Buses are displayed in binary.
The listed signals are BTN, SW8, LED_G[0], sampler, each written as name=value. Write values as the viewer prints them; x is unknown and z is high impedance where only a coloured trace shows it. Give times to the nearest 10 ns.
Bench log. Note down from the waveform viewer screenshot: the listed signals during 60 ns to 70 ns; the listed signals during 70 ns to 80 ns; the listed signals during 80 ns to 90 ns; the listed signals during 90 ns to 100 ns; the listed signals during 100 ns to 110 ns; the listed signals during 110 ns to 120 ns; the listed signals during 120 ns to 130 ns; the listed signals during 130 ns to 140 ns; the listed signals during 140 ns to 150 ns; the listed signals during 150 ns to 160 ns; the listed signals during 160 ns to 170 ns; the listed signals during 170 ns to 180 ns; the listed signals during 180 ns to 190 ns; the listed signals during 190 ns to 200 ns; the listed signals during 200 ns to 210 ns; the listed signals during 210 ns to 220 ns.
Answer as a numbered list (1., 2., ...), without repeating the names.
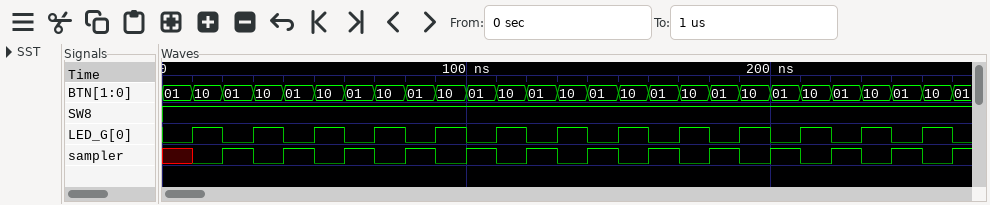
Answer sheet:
1. BTN=01, SW8=1, LED_G[0]=0, sampler=1
2. BTN=10, SW8=1, LED_G[0]=1, sampler=0
3. BTN=01, SW8=1, LED_G[0]=0, sampler=1
4. BTN=10, SW8=1, LED_G[0]=1, sampler=0
5. BTN=01, SW8=1, LED_G[0]=0, sampler=1
6. BTN=10, SW8=1, LED_G[0]=1, sampler=0
7. BTN=01, SW8=1, LED_G[0]=0, sampler=1
8. BTN=10, SW8=1, LED_G[0]=1, sampler=0
9. BTN=01, SW8=1, LED_G[0]=0, sampler=1
10. BTN=10, SW8=1, LED_G[0]=1, sampler=0
11. BTN=01, SW8=1, LED_G[0]=0, sampler=1
12. BTN=10, SW8=1, LED_G[0]=1, sampler=0
13. BTN=01, SW8=1, LED_G[0]=0, sampler=1
14. BTN=10, SW8=1, LED_G[0]=1, sampler=0
15. BTN=01, SW8=1, LED_G[0]=0, sampler=1
16. BTN=10, SW8=1, LED_G[0]=1, sampler=0
